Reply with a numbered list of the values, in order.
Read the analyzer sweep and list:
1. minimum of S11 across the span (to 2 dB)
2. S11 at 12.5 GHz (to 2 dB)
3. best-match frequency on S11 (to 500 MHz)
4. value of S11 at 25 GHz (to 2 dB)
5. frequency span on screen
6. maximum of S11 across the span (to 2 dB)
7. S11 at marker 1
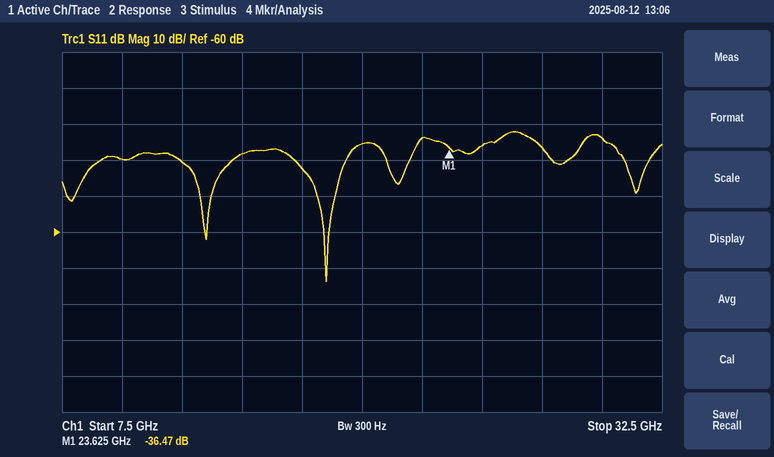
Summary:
1. -74 dB
2. -40 dB
3. 18.5 GHz
4. -36 dB
5. 25 GHz
6. -32 dB
7. -36.47 dB
